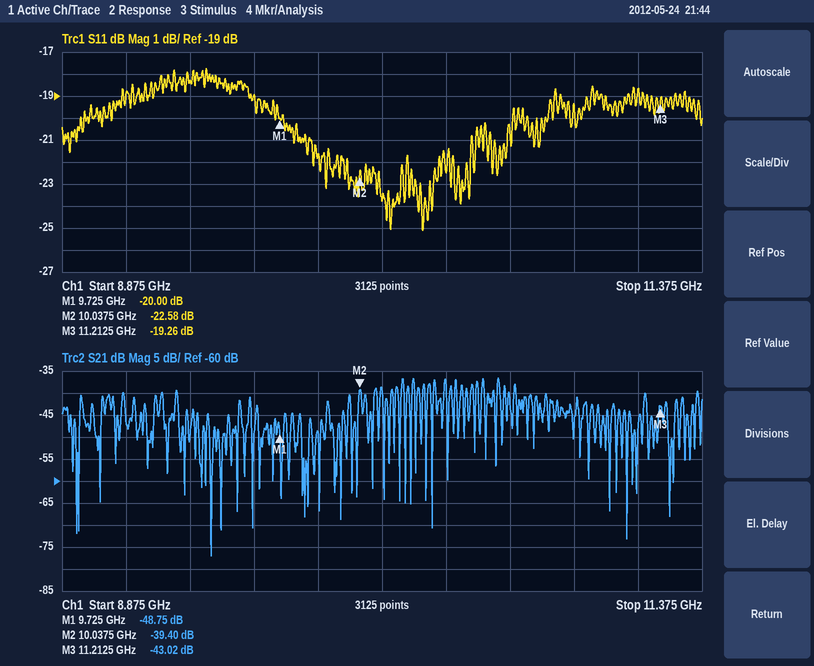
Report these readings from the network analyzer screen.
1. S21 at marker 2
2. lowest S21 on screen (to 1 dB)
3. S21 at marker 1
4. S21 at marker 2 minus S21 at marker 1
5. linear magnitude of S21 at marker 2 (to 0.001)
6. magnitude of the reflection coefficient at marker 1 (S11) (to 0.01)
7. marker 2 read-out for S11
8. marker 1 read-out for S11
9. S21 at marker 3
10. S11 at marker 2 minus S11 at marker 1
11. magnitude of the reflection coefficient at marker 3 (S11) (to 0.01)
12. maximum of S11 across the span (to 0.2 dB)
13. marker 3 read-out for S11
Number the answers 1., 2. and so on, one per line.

1. -39.40 dB
2. -77 dB
3. -48.75 dB
4. 9.35 dB
5. 0.011
6. 0.10
7. -22.58 dB
8. -20.00 dB
9. -43.02 dB
10. -2.58 dB
11. 0.11
12. -17.8 dB
13. -19.26 dB
